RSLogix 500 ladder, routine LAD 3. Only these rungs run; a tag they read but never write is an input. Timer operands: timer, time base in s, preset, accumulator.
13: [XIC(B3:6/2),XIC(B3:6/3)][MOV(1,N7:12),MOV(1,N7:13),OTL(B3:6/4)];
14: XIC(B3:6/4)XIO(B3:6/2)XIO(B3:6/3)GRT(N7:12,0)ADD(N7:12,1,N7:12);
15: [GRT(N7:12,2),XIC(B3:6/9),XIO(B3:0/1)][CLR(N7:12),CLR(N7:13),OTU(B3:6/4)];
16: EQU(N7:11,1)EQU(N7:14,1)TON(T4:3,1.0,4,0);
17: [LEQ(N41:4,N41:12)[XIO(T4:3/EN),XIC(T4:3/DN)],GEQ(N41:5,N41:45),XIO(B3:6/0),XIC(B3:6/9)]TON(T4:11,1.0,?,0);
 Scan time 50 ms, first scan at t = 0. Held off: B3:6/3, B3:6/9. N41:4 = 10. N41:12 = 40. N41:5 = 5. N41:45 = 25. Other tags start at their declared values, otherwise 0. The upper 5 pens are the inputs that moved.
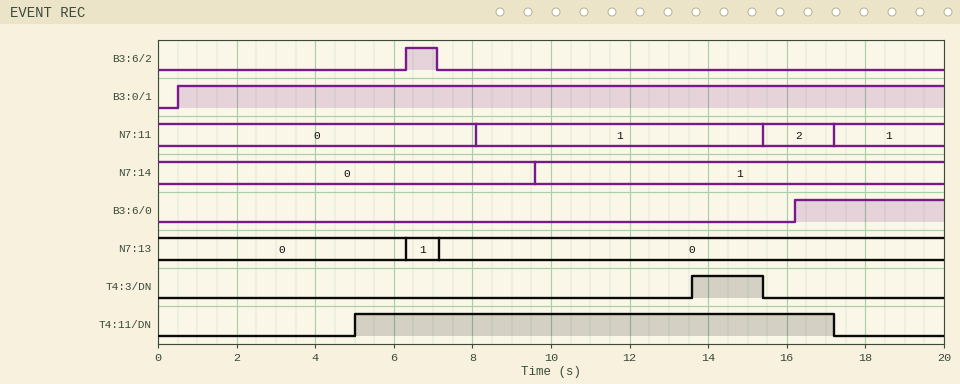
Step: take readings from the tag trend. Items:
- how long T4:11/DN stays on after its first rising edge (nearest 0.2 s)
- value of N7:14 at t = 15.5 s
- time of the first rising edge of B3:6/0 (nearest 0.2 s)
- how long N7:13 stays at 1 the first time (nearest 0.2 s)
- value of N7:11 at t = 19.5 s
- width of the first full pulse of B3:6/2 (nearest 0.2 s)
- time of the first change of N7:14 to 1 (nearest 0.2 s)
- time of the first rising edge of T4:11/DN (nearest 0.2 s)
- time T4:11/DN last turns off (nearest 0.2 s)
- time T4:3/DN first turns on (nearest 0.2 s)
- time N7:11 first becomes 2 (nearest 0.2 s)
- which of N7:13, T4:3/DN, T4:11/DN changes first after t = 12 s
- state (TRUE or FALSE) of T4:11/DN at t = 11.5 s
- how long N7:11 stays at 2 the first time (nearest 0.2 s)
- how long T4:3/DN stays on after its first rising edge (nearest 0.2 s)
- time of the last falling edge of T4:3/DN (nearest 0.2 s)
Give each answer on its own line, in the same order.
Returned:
12.2 s
1
16.2 s
0.8 s
1
0.8 s
9.6 s
5.0 s
17.2 s
13.6 s
15.4 s
T4:3/DN
TRUE
1.8 s
1.8 s
15.4 s
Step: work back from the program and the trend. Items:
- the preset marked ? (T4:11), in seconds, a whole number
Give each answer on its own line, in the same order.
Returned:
5 s
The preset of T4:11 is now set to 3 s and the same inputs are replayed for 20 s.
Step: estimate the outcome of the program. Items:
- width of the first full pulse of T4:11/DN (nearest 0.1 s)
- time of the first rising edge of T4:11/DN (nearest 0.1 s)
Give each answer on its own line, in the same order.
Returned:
14.2 s
3.0 s
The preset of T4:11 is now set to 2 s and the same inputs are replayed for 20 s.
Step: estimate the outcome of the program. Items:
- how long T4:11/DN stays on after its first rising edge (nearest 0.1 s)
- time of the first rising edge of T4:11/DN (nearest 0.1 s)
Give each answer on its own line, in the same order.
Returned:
15.2 s
2.0 s
